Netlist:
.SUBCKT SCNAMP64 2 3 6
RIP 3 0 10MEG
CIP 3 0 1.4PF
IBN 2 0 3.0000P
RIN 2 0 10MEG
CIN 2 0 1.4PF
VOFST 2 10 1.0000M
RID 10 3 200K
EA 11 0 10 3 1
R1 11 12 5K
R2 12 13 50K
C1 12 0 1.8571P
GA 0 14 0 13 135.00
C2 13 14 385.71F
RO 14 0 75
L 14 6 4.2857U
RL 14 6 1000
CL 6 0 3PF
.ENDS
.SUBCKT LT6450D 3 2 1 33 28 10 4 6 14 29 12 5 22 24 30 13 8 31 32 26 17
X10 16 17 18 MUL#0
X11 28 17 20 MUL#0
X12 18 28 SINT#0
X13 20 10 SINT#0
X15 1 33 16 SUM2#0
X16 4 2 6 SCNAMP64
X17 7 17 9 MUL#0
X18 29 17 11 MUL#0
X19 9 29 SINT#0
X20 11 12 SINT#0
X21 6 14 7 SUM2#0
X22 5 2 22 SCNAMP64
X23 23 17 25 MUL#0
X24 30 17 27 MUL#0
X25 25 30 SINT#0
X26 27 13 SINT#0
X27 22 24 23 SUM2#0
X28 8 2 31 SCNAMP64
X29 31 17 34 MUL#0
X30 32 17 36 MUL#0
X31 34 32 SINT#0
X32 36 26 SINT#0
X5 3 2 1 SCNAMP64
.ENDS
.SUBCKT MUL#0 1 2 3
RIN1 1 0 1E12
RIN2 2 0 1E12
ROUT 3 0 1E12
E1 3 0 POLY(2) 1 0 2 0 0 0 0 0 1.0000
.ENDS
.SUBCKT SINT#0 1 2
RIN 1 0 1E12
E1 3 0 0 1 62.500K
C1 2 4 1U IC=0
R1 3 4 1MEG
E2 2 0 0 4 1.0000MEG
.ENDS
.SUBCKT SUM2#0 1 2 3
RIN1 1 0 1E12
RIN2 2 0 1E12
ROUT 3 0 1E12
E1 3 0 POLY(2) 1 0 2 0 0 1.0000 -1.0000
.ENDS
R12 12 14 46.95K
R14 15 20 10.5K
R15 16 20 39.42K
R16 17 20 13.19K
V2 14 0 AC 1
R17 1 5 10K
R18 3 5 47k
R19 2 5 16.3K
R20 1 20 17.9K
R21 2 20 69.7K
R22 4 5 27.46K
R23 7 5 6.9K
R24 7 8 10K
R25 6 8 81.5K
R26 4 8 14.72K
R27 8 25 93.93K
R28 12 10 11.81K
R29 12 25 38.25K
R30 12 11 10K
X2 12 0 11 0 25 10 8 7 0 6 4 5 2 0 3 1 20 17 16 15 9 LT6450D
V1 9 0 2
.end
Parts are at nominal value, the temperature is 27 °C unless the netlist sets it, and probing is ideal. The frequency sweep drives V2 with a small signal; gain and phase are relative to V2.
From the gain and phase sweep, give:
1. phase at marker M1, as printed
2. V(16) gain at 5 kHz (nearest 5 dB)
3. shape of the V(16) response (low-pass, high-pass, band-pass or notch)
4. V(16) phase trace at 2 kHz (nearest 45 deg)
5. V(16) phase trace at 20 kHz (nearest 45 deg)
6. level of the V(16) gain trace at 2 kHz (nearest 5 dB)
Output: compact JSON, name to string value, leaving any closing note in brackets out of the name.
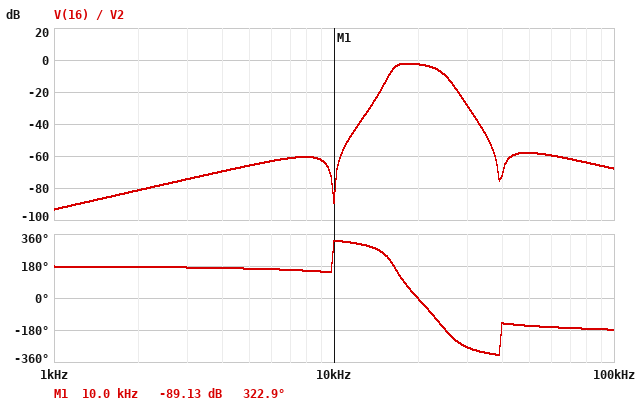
{"phase at marker M1, as printed": "322.9 deg", "V(16) gain at 5 kHz": "-65 dB", "shape of the V(16) response": "band-pass", "V(16) phase trace at 2 kHz": "180 deg", "V(16) phase trace at 20 kHz": "0 deg", "level of the V(16) gain trace at 2 kHz": "-80 dB"}
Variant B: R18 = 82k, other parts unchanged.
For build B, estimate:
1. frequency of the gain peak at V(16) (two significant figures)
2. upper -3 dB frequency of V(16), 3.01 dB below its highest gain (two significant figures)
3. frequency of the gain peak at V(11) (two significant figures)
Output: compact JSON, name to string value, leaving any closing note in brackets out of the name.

{"frequency of the gain peak at V(16)": "19 kHz", "upper -3 dB frequency of V(16), 3.01 dB below its highest gain": "25 kHz", "frequency of the gain peak at V(11)": "19 kHz"}
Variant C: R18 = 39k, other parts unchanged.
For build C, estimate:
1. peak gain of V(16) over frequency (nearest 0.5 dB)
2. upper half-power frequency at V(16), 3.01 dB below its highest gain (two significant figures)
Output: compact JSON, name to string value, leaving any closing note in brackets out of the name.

{"peak gain of V(16) over frequency": "-2.5 dB", "upper half-power frequency at V(16), 3.01 dB below its highest gain": "22 kHz"}
